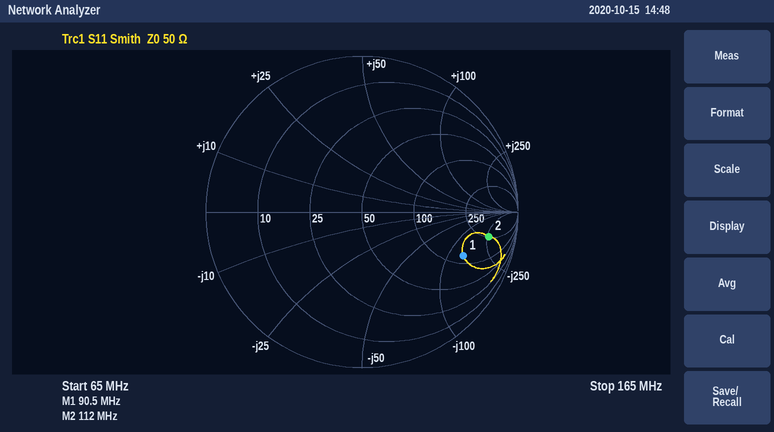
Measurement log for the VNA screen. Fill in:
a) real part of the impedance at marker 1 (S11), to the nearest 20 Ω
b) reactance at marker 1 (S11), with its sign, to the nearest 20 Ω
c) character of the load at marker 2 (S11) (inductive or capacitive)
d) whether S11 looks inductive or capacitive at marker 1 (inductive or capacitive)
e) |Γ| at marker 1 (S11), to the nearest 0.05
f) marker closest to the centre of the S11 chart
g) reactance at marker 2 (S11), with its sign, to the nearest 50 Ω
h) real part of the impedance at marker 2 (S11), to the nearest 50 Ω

120 Ω
-140 Ω
capacitive
capacitive
0.70
marker 1
-250 Ω
250 Ω
